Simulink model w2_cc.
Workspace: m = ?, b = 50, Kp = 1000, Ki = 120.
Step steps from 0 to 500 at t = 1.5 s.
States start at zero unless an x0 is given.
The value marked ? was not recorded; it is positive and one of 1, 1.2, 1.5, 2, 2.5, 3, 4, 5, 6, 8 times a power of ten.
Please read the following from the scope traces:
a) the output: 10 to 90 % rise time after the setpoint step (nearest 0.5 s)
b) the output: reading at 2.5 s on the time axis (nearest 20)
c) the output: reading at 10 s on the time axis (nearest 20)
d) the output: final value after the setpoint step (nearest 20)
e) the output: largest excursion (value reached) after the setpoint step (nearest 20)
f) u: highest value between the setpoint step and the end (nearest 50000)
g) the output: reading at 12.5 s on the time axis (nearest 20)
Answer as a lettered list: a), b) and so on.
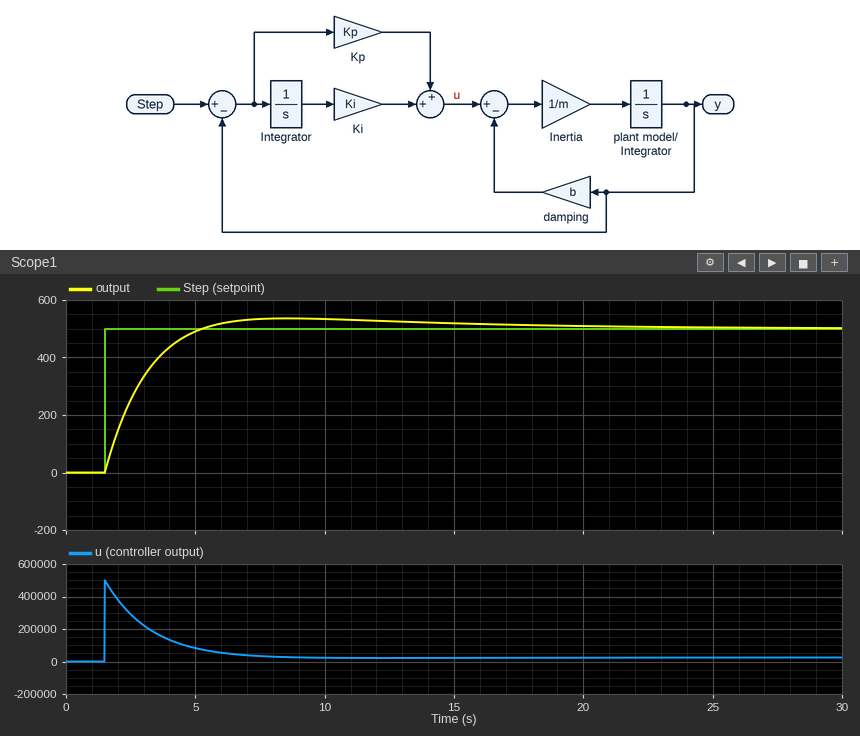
a) 2.5 s
b) 260
c) 540
d) 500
e) 540
f) 500000
g) 520
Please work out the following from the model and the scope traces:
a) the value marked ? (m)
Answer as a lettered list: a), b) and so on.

a) 1500
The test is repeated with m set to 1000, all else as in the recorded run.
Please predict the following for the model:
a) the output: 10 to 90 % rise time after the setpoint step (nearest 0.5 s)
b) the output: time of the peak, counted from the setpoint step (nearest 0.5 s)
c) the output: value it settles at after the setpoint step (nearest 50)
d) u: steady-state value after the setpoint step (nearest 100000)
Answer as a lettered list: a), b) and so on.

a) 2.0 s
b) 5.5 s
c) 500
d) 0
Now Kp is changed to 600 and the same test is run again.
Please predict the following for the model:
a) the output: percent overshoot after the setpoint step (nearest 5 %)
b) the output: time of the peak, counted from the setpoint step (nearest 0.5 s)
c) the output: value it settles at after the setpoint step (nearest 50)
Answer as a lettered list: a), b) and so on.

a) 15 %
b) 8.0 s
c) 500
